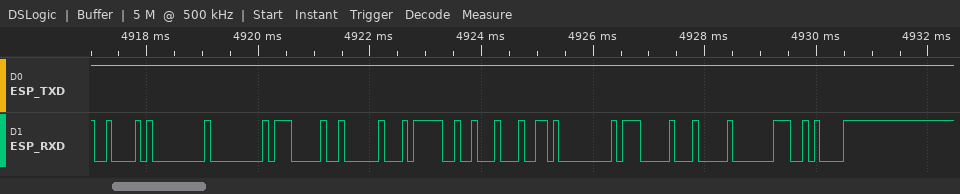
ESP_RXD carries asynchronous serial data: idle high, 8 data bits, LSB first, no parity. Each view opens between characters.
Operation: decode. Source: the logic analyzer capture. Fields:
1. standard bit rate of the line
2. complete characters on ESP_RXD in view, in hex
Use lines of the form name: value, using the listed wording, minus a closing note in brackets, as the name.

standard bit rate of the line: 9600 baud
complete characters on ESP_RXD in view, in hex: 42, 00, 00, 07, 02, F4, 12, 64, 00, 07, 04, C0, 0A
